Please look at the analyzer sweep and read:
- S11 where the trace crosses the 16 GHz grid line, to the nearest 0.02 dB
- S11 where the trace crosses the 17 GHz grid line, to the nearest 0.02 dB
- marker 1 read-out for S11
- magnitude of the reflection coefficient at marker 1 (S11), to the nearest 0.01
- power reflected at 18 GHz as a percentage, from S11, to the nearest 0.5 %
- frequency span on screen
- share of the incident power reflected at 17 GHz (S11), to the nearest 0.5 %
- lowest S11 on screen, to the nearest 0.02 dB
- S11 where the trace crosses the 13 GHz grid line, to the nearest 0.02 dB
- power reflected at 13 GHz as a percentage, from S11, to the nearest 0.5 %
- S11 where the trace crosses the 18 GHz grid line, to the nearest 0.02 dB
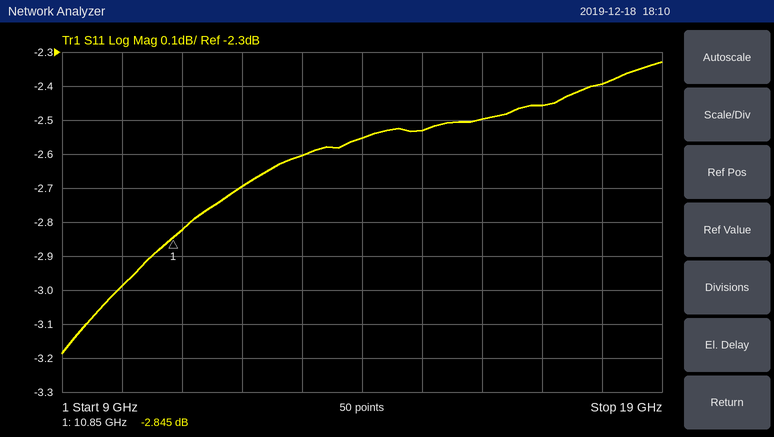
-2.50 dB
-2.46 dB
-2.845 dB
0.72
57.5 %
10 GHz
57.0 %
-3.18 dB
-2.60 dB
55.0 %
-2.40 dB
